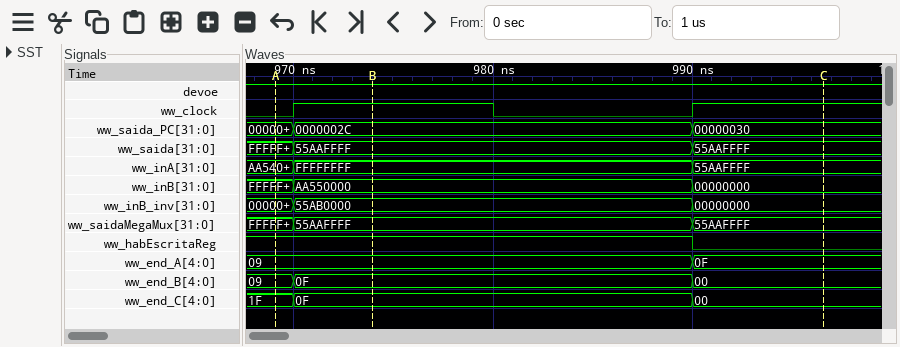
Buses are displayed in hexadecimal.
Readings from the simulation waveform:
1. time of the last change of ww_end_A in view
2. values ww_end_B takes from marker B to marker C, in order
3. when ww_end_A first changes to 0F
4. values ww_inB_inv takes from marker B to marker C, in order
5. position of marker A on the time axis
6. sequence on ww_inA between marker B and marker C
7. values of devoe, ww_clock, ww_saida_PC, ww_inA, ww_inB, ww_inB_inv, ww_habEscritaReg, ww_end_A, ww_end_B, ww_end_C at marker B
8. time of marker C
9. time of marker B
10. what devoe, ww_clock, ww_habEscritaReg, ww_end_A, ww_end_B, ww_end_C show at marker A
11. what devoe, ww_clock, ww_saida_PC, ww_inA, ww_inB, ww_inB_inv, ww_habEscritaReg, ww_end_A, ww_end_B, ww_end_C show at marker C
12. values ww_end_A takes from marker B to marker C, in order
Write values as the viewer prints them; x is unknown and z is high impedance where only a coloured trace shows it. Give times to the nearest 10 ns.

990 ns
0F, 00
990 ns
55AB0000, 00000000
970 ns
FFFFFFFF, 55AAFFFF
devoe=1, ww_clock=1, ww_saida_PC=0000002C, ww_inA=FFFFFFFF, ww_inB=AA550000, ww_inB_inv=55AB0000, ww_habEscritaReg=1, ww_end_A=09, ww_end_B=0F, ww_end_C=0F
1000 ns
970 ns
devoe=1, ww_clock=0, ww_habEscritaReg=1, ww_end_A=09, ww_end_B=09, ww_end_C=1F
devoe=1, ww_clock=1, ww_saida_PC=00000030, ww_inA=55AAFFFF, ww_inB=00000000, ww_inB_inv=00000000, ww_habEscritaReg=0, ww_end_A=0F, ww_end_B=00, ww_end_C=00
09, 0F
